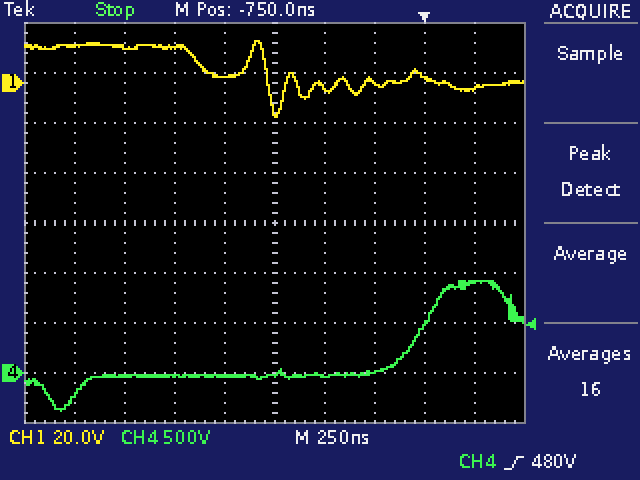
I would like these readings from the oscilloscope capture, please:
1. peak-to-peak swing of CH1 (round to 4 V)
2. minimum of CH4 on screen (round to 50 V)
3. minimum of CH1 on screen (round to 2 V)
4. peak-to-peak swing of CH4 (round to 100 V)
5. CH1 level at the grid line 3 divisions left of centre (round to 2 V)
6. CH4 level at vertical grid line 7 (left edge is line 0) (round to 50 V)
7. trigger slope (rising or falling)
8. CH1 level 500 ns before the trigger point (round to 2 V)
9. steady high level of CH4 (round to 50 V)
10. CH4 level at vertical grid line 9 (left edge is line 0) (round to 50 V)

32 V
-400 V
-14 V
1.30 kV
14 V
0 V
rising
-2 V
900 V
900 V
